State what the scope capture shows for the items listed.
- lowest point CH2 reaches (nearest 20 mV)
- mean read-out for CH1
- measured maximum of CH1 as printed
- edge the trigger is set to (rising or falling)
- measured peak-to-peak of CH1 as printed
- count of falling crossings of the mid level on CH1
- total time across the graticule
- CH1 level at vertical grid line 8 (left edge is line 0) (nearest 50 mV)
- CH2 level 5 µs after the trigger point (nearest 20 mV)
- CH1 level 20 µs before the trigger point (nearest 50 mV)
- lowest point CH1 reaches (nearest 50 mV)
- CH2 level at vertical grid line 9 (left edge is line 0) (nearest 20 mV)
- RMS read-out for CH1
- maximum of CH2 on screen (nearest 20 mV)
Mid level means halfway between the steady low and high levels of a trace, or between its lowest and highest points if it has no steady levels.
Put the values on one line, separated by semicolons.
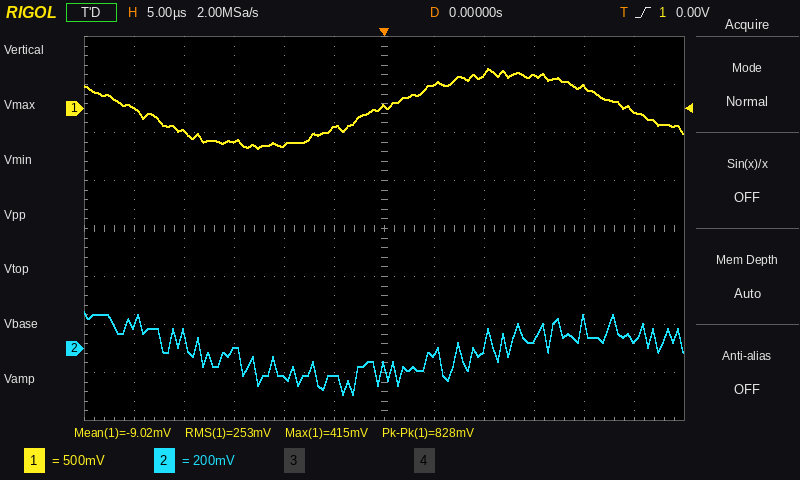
-200 mV; -9.02 mV; 415 mV; rising; 828 mV; 2; 60 µs; 350 mV; -20 mV; -250 mV; -400 mV; 40 mV; 253 mV; 160 mV
